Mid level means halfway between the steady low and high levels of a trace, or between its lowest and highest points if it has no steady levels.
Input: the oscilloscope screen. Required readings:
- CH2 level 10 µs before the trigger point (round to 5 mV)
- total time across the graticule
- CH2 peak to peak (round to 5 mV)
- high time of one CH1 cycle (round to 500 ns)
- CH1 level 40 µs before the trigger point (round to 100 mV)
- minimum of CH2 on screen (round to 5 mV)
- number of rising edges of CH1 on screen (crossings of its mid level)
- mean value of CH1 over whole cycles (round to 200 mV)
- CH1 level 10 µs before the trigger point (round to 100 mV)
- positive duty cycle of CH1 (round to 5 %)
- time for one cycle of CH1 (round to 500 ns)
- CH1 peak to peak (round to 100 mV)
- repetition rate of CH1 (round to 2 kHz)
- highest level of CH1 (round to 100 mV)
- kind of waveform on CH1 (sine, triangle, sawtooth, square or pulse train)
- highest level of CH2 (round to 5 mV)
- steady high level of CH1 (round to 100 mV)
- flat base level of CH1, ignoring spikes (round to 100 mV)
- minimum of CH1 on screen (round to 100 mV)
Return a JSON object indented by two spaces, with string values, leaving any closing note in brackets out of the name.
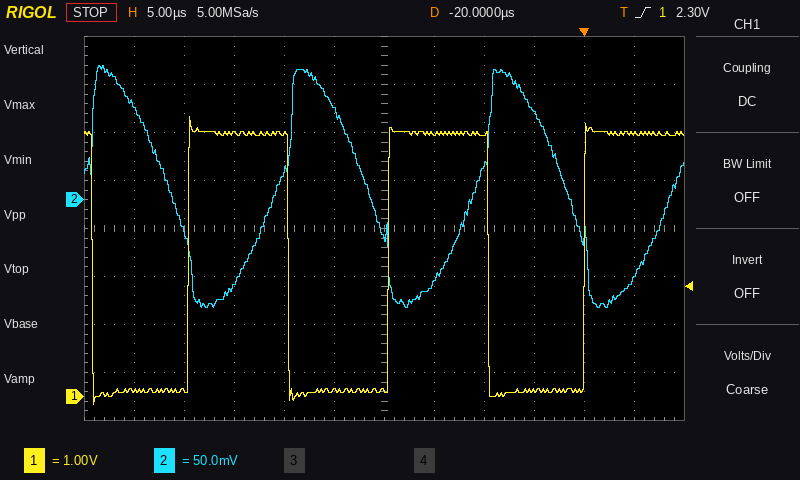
{
  "CH2 level 10 µs before the trigger point": "35 mV",
  "total time across the graticule": "60 µs",
  "CH2 peak to peak": "250 mV",
  "high time of one CH1 cycle": "10.0 µs",
  "CH1 level 40 µs before the trigger point": "100 mV",
  "minimum of CH2 on screen": "-110 mV",
  "number of rising edges of CH1 on screen": "3",
  "mean value of CH1 over whole cycles": "2.8 V",
  "CH1 level 10 µs before the trigger point": "5.5 V",
  "positive duty cycle of CH1": "50 %",
  "time for one cycle of CH1": "20.0 µs",
  "CH1 peak to peak": "6.0 V",
  "repetition rate of CH1": "50 kHz",
  "highest level of CH1": "5.8 V",
  "kind of waveform on CH1": "square",
  "highest level of CH2": "140 mV",
  "steady high level of CH1": "5.5 V",
  "flat base level of CH1, ignoring spikes": "100 mV",
  "minimum of CH1 on screen": "-200 mV"
}
